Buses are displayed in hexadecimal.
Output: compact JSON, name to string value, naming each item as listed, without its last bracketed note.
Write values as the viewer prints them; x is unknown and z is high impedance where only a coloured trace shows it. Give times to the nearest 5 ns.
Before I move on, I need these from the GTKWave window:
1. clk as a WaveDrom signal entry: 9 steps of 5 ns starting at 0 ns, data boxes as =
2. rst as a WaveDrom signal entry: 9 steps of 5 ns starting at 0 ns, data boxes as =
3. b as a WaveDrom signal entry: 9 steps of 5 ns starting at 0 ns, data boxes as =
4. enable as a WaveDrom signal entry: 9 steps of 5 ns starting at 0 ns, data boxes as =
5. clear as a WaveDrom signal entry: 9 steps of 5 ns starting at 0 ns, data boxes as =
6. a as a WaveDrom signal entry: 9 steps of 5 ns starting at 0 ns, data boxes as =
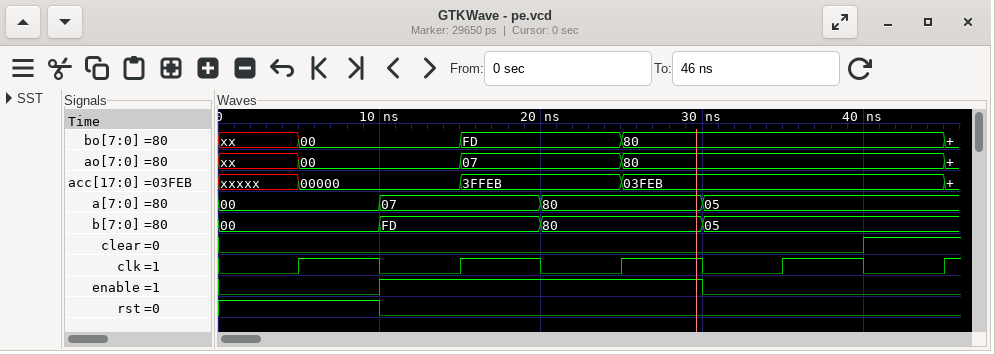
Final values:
{"clk as a WaveDrom signal entry: 9 steps of 5 ns starting at 0 ns, data boxes as =": "{name: 'clk', wave: '010101010'}", "rst as a WaveDrom signal entry: 9 steps of 5 ns starting at 0 ns, data boxes as =": "{name: 'rst', wave: '1.0......'}", "b as a WaveDrom signal entry: 9 steps of 5 ns starting at 0 ns, data boxes as =": "{name: 'b', wave: '=.=.=.=..', data: '00 FD 80 05'}", "enable as a WaveDrom signal entry: 9 steps of 5 ns starting at 0 ns, data boxes as =": "{name: 'enable', wave: '0.1...0..'}", "clear as a WaveDrom signal entry: 9 steps of 5 ns starting at 0 ns, data boxes as =": "{name: 'clear', wave: '0.......1'}", "a as a WaveDrom signal entry: 9 steps of 5 ns starting at 0 ns, data boxes as =": "{name: 'a', wave: '=.=.=.=..', data: '00 07 80 05'}"}
